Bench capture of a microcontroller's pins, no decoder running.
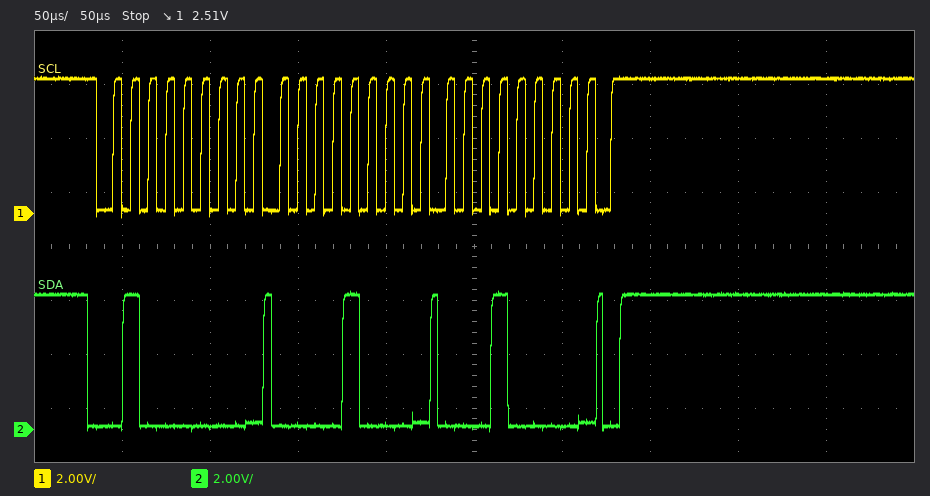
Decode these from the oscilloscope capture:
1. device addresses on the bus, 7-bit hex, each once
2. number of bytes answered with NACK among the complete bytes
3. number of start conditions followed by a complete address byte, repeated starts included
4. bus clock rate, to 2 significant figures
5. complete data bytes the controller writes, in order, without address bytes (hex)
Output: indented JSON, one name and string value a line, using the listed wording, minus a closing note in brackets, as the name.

{
  "device addresses on the bus, 7-bit hex, each once": "0x20",
  "number of bytes answered with NACK among the complete bytes": "0",
  "number of start conditions followed by a complete address byte, repeated starts included": "1",
  "bus clock rate, to 2 significant figures": "100 kHz",
  "complete data bytes the controller writes, in order, without address bytes": "08 10"
}
